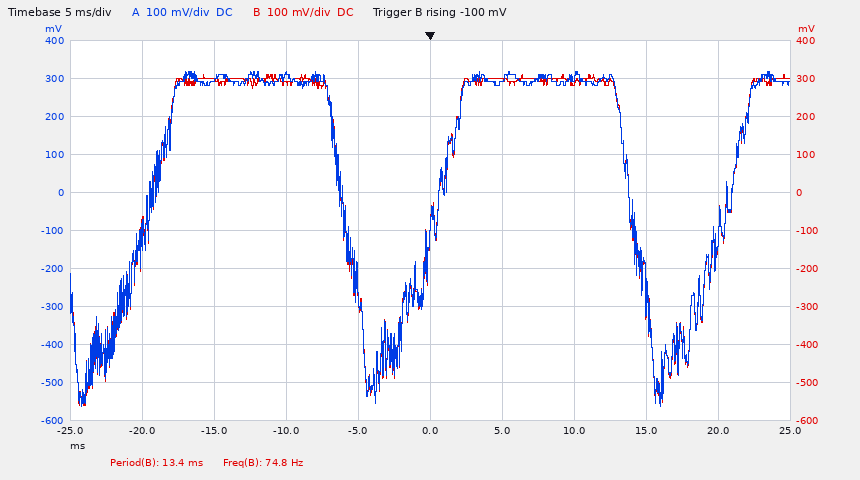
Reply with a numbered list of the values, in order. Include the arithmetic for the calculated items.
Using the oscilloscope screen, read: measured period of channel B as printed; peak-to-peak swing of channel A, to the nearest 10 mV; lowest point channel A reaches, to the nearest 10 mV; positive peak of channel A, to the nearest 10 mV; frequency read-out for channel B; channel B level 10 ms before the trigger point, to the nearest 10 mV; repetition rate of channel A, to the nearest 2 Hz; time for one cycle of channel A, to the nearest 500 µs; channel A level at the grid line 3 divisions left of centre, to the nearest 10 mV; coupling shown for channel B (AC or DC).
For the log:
1. 13.4 ms
2. 320 mV − (-560 mV) = 880 mV
3. -560 mV
4. 320 mV
5. 74.8 Hz
6. 290 mV
7. 1 / 20.0 ms ≈ 50 Hz
8. 20.0 ms
9. 300 mV
10. DC
